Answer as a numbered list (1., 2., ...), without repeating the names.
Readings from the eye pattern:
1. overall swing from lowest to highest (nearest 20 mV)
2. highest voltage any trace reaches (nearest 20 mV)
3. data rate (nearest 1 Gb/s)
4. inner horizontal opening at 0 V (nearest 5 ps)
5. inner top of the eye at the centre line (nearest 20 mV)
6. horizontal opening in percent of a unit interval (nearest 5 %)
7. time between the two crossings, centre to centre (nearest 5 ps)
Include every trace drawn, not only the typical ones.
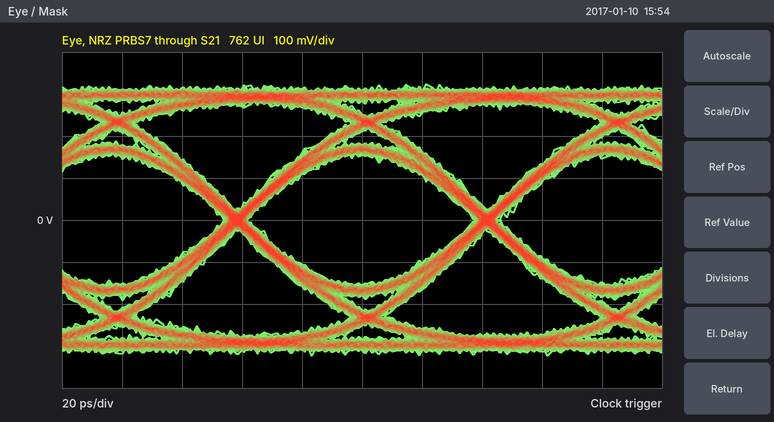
1. 640 mV
2. 320 mV
3. 12 Gb/s
4. 75 ps
5. 160 mV
6. 90 %
7. 85 ps
